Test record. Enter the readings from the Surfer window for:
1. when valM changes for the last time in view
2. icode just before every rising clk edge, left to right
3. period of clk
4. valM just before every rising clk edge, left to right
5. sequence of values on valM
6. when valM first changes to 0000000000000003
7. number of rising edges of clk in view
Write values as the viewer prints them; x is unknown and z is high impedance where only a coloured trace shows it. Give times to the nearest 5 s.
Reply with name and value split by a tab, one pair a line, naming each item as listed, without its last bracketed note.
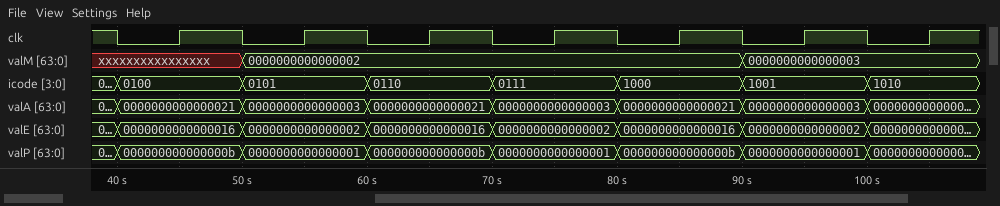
when valM changes for the last time in view	90 s
icode just before every rising clk edge, left to right	0100, 0101, 0110, 0111, 1000, 1001, 1010
period of clk	10 s
valM just before every rising clk edge, left to right	xxxxxxxxxxxxxxxx, 0000000000000002, 0000000000000002, 0000000000000002, 0000000000000002, 0000000000000003, 0000000000000003
sequence of values on valM	xxxxxxxxxxxxxxxx, 0000000000000002, 0000000000000003
when valM first changes to 0000000000000003	90 s
number of rising edges of clk in view	7
